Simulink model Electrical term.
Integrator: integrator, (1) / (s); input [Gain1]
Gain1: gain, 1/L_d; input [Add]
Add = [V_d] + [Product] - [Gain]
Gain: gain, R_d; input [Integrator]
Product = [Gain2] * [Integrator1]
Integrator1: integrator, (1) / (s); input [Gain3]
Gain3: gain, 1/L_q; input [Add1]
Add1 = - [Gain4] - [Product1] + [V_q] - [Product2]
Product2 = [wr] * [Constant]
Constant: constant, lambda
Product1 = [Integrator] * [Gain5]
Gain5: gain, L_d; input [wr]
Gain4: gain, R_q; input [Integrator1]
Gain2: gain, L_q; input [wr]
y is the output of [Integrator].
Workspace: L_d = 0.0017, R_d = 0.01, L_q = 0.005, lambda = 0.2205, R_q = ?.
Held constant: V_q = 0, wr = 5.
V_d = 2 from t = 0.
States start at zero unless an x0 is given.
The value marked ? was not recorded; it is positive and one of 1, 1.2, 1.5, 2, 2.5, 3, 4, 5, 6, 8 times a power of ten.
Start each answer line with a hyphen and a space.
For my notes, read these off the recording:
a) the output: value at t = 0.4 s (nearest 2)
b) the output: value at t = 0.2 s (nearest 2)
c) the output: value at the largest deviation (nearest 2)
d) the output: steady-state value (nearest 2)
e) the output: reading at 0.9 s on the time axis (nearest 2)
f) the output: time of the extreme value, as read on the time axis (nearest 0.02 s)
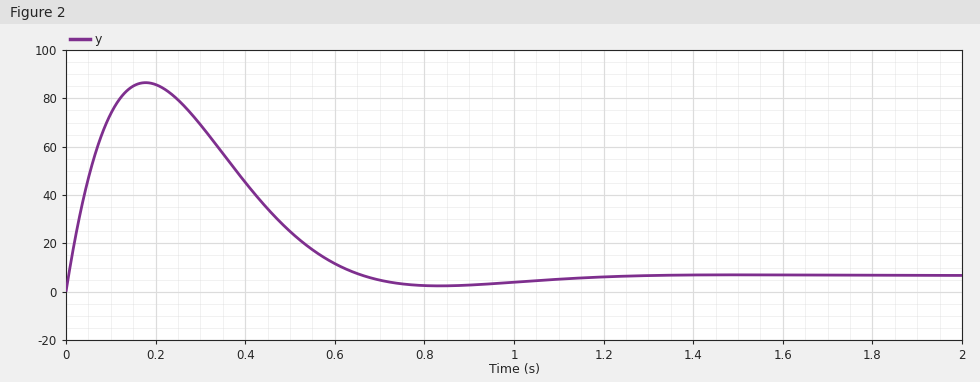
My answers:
- 46
- 86
- 86
- 6
- 2
- 0.18 s
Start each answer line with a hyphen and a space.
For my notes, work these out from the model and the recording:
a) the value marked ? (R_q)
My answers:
- 0.015
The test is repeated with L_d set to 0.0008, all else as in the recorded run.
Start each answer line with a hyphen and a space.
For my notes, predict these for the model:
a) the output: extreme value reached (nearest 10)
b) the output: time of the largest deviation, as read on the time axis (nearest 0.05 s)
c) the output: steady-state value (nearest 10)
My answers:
- 120
- 0.15 s
- 10
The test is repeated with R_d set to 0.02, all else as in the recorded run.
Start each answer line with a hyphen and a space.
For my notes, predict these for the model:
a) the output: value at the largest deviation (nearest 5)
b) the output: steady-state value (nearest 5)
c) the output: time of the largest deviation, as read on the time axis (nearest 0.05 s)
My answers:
- 60
- 5
- 0.15 s
